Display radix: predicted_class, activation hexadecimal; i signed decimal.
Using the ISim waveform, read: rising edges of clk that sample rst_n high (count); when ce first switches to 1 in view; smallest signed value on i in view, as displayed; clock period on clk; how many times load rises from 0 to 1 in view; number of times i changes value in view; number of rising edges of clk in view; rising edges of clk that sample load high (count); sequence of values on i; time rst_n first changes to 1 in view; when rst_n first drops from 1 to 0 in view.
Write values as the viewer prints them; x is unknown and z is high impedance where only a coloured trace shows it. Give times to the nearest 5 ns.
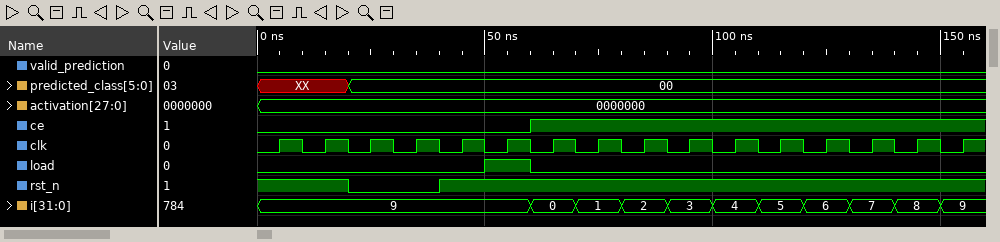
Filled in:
14
60 ns
0
10 ns
1
10
16
1
9, 0, 1, 2, 3, 4, 5, 6, 7, 8, 9
40 ns
20 ns
